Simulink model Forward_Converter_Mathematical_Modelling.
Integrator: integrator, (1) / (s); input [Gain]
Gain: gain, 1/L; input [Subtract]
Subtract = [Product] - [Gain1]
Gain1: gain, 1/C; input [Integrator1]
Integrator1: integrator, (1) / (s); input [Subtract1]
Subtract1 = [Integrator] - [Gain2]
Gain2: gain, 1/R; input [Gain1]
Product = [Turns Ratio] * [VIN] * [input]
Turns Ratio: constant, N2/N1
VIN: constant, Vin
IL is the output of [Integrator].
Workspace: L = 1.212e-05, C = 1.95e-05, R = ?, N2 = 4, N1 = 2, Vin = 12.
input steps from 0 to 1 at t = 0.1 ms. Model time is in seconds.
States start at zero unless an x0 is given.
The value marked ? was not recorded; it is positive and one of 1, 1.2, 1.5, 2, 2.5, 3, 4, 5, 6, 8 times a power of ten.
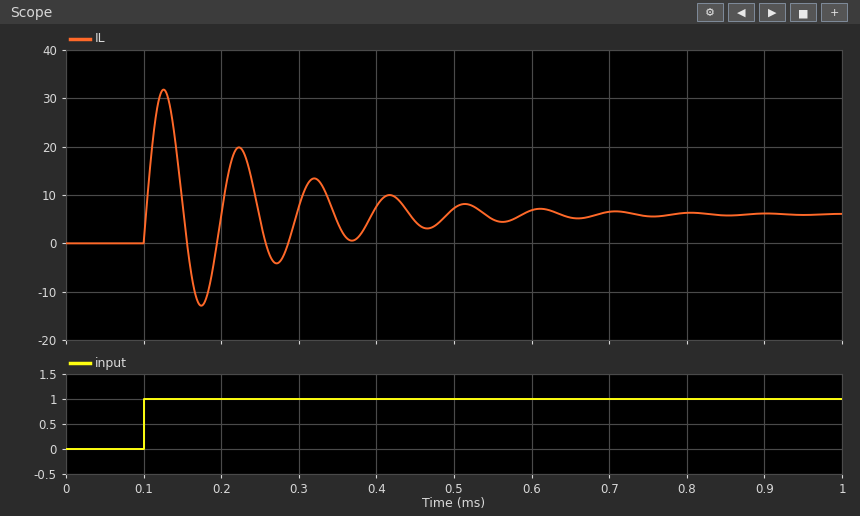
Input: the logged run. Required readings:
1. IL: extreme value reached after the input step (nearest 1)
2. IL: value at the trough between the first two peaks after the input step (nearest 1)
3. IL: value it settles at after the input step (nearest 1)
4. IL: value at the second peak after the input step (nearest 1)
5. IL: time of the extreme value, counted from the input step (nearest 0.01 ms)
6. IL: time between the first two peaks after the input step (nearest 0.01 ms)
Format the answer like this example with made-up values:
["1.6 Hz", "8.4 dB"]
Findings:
["32", "-13", "6", "20", "0.03 ms", "0.10 ms"]
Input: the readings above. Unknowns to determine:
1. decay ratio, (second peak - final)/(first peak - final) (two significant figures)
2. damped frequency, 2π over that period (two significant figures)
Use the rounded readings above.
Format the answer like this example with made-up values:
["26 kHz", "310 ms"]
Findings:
["0.54", "63 rad/ms"]
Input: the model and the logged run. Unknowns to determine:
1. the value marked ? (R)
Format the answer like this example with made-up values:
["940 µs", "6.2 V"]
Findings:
["4"]
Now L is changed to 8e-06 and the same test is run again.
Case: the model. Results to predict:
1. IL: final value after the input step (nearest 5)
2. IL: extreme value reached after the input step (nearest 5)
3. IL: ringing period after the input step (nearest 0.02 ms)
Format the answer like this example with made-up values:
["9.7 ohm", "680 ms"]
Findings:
["5", "40", "0.08 ms"]
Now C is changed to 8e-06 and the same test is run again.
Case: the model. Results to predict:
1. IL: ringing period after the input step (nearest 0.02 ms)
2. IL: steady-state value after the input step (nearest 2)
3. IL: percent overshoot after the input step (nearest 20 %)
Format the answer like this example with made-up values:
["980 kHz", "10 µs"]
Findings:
["0.06 ms", "6", "240 %"]
